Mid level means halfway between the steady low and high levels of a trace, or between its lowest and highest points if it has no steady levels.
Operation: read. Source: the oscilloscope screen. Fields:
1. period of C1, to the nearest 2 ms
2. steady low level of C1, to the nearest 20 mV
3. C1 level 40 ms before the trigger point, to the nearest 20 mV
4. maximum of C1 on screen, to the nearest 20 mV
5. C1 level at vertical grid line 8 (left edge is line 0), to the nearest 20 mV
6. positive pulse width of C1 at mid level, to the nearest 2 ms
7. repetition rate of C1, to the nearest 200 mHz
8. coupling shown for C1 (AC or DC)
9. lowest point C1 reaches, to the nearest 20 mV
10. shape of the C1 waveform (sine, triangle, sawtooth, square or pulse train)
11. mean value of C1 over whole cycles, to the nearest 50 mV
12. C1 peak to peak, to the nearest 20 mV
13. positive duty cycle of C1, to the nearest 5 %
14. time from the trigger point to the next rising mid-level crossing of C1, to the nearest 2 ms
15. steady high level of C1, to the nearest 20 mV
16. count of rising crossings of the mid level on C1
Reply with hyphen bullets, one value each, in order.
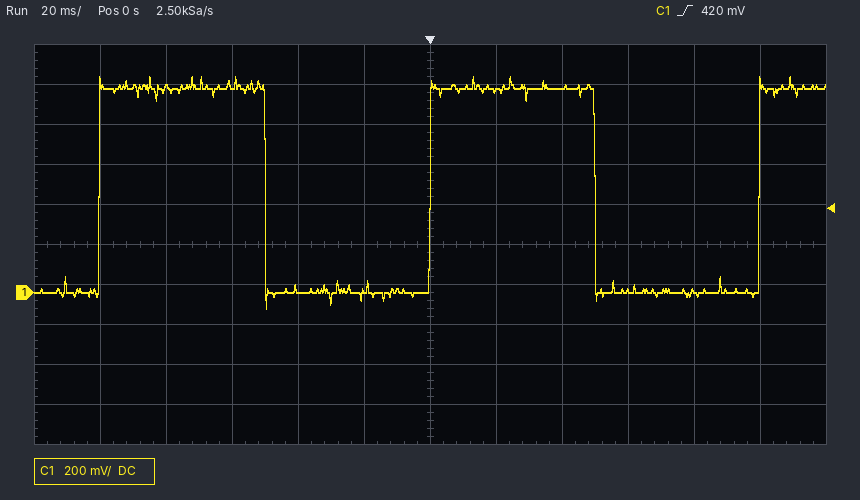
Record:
- 100 ms
- 0 mV
- 20 mV
- 1.08 V
- 1.02 V
- 50 ms
- 10.0 Hz
- DC
- -80 mV
- square
- 500 mV
- 1.16 V
- 50 %
- 100 ms
- 1.02 V
- 3
